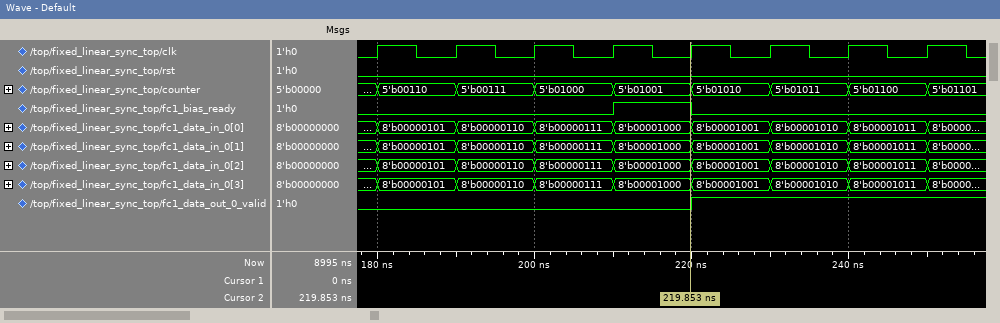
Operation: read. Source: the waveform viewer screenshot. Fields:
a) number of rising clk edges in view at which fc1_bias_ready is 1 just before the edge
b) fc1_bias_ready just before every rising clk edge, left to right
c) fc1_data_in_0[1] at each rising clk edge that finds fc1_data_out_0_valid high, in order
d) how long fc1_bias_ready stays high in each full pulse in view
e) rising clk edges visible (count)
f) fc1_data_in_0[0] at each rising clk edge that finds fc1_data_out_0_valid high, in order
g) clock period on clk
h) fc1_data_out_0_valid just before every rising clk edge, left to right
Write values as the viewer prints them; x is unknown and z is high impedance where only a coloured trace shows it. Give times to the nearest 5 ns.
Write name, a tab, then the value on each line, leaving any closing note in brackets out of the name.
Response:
number of rising clk edges in view at which fc1_bias_ready is 1 just before the edge	1
fc1_bias_ready just before every rising clk edge, left to right	0 0 0 0 1 0 0 0
fc1_data_in_0[1] at each rising clk edge that finds fc1_data_out_0_valid high, in order	8'b00001001, 8'b00001010, 8'b00001011
how long fc1_bias_ready stays high in each full pulse in view	10 ns
rising clk edges visible	8
fc1_data_in_0[0] at each rising clk edge that finds fc1_data_out_0_valid high, in order	8'b00001001, 8'b00001010, 8'b00001011
clock period on clk	10 ns
fc1_data_out_0_valid just before every rising clk edge, left to right	0 0 0 0 0 1 1 1
